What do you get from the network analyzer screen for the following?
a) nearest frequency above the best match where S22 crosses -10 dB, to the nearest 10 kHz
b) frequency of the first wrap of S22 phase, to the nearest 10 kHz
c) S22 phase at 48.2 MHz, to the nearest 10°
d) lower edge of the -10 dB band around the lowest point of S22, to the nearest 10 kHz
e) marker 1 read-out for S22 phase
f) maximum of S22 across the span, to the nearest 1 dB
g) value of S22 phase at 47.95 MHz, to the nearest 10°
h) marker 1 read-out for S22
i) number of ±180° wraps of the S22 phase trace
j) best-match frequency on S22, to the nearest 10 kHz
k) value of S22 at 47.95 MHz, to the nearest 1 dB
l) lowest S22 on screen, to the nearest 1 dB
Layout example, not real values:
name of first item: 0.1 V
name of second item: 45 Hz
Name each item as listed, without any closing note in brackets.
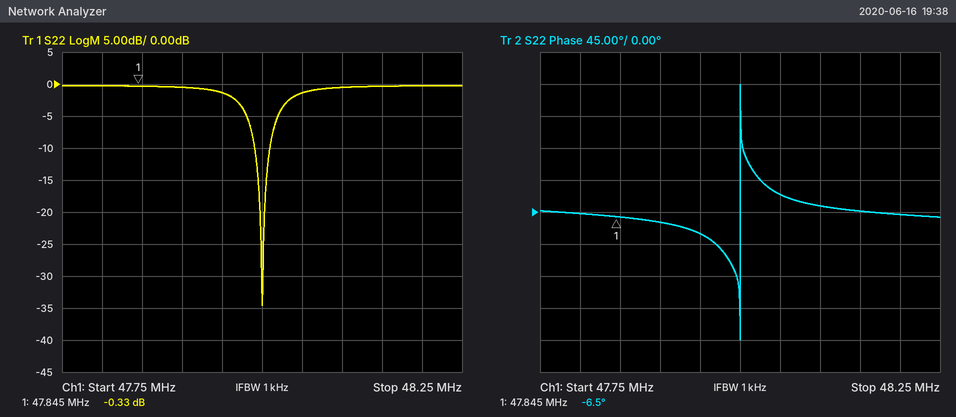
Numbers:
nearest frequency above the best match where S22 crosses -10 dB, to the nearest 10 kHz: 48.01 MHz
frequency of the first wrap of S22 phase, to the nearest 10 kHz: 48.00 MHz
S22 phase at 48.2 MHz, to the nearest 10°: 0°
lower edge of the -10 dB band around the lowest point of S22, to the nearest 10 kHz: 47.99 MHz
marker 1 read-out for S22 phase: -6.5°
maximum of S22 across the span, to the nearest 1 dB: 0 dB
value of S22 phase at 47.95 MHz, to the nearest 10°: -30°
marker 1 read-out for S22: -0.33 dB
number of ±180° wraps of the S22 phase trace: 1
best-match frequency on S22, to the nearest 10 kHz: 48.00 MHz
value of S22 at 47.95 MHz, to the nearest 1 dB: -1 dB
lowest S22 on screen, to the nearest 1 dB: -35 dB
